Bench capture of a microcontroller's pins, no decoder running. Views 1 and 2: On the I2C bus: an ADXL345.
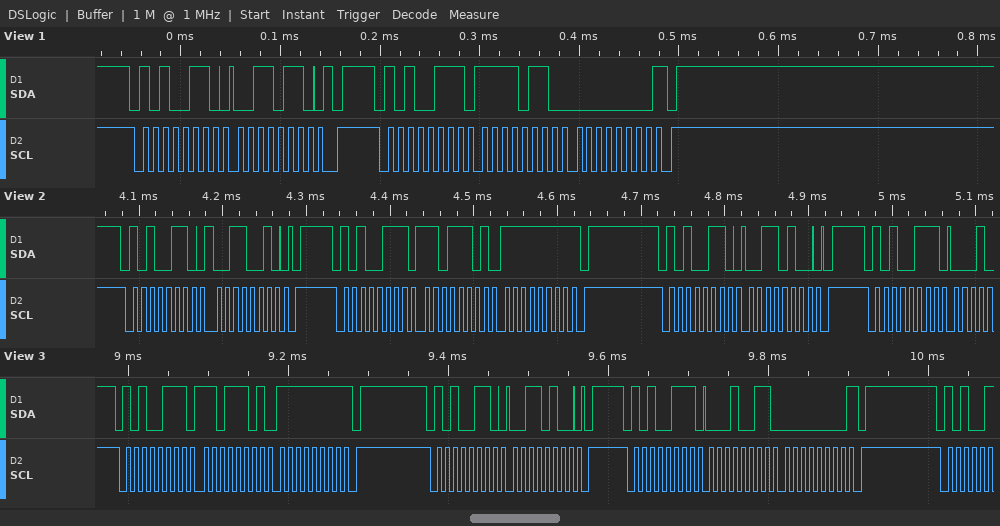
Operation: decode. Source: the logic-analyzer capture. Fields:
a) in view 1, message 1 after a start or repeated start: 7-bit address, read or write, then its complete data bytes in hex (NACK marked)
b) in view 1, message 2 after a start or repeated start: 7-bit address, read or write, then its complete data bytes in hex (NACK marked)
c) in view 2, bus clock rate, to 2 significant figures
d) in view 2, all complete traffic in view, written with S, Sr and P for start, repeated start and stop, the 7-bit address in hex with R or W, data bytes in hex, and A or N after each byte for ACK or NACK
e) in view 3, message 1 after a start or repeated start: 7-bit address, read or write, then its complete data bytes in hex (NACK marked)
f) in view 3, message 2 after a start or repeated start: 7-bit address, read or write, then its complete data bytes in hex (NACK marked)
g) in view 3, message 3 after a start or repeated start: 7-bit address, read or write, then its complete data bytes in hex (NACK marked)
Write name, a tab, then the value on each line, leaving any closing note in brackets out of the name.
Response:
in view 1, message 1 after a start or repeated start: 7-bit address, read or write, then its complete data bytes in hex	0x53 write: 36
in view 1, message 2 after a start or repeated start: 7-bit address, read or write, then its complete data bytes in hex	0x53 read: F6 00 NACK
in view 2, bus clock rate, to 2 significant figures	100 kHz
in view 2, all complete traffic in view, written with S, Sr and P for start, repeated start and stop, the 7-bit address in hex with R or W, data bytes in hex, and A or N after each byte for ACK or NACK	S 53W A 32 A P S 53R A DD A FF N P S 53W A 34 A P S 53R A
in view 3, message 1 after a start or repeated start: 7-bit address, read or write, then its complete data bytes in hex	0x53 read: DD FF NACK
in view 3, message 2 after a start or repeated start: 7-bit address, read or write, then its complete data bytes in hex	0x53 write: 34
in view 3, message 3 after a start or repeated start: 7-bit address, read or write, then its complete data bytes in hex	0x53 read: 13 00 NACK
